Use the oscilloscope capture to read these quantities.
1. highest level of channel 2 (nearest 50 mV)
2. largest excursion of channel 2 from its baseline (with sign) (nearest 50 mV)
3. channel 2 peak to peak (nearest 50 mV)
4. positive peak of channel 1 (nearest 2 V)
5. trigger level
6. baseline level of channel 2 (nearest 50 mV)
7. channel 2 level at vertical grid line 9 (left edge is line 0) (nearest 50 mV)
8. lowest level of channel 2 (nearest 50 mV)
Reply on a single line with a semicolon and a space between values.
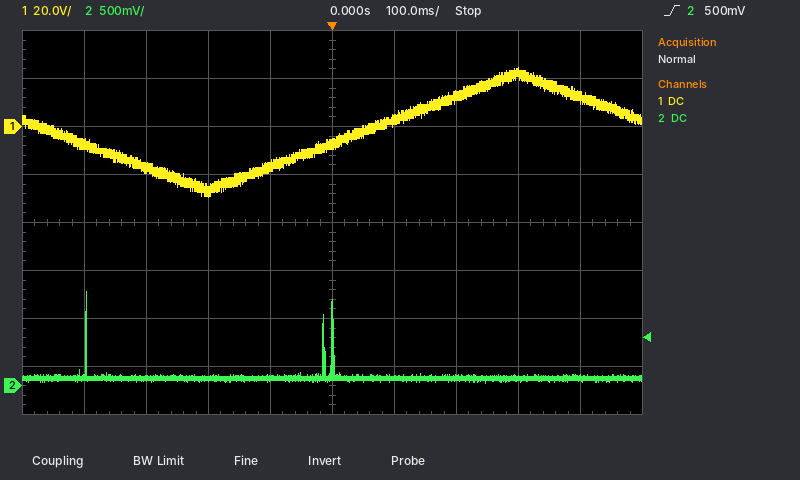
1.00 V; +900 mV; 950 mV; 24 V; 500 mV; 100 mV; 100 mV; 50 mV
